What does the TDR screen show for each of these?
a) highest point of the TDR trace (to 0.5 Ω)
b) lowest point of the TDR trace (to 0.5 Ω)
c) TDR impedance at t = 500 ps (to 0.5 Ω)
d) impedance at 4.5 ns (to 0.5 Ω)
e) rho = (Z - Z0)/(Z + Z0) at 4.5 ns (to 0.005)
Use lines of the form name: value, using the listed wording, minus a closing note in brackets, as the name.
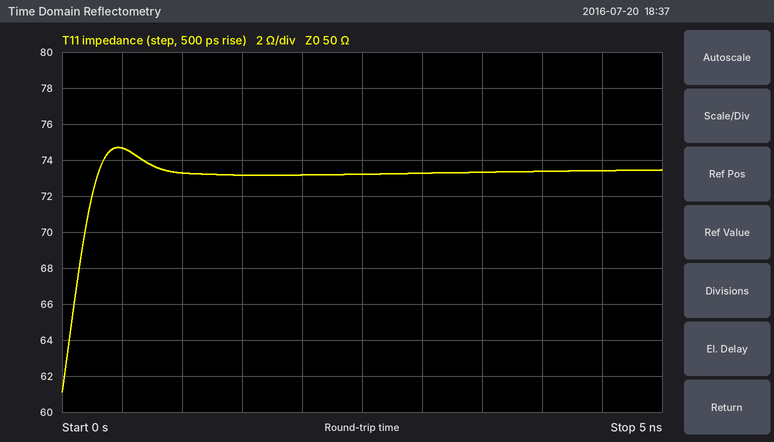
highest point of the TDR trace: 74.5 Ω
lowest point of the TDR trace: 61.0 Ω
TDR impedance at t = 500 ps: 74.5 Ω
impedance at 4.5 ns: 73.5 Ω
rho = (Z - Z0)/(Z + Z0) at 4.5 ns: +0.190
